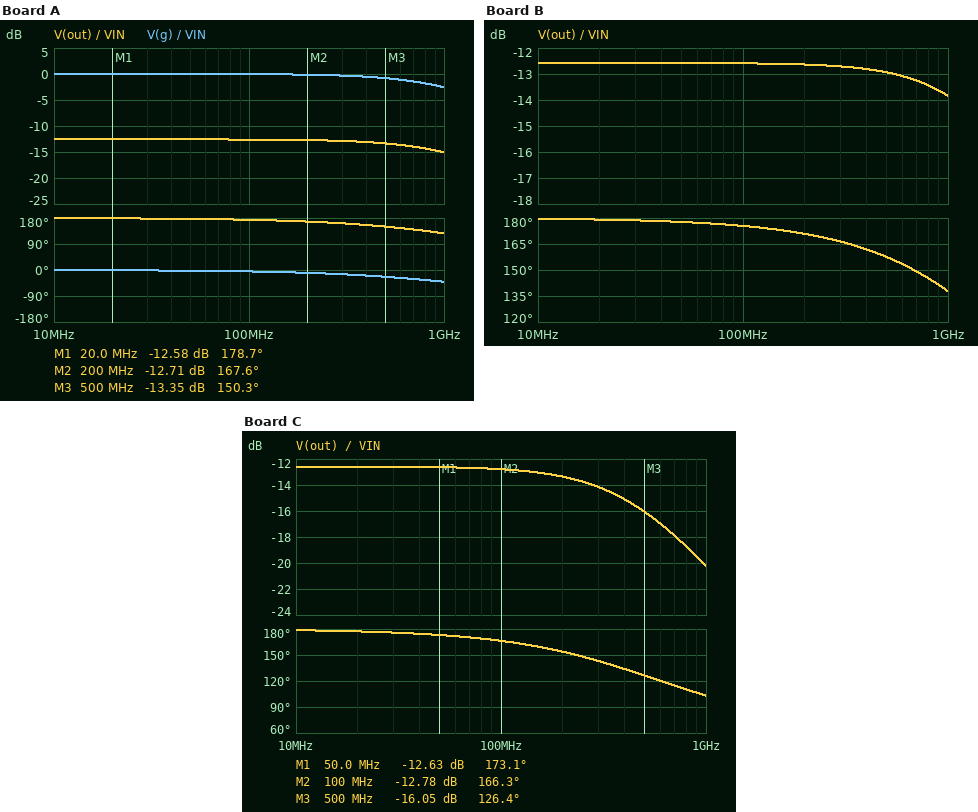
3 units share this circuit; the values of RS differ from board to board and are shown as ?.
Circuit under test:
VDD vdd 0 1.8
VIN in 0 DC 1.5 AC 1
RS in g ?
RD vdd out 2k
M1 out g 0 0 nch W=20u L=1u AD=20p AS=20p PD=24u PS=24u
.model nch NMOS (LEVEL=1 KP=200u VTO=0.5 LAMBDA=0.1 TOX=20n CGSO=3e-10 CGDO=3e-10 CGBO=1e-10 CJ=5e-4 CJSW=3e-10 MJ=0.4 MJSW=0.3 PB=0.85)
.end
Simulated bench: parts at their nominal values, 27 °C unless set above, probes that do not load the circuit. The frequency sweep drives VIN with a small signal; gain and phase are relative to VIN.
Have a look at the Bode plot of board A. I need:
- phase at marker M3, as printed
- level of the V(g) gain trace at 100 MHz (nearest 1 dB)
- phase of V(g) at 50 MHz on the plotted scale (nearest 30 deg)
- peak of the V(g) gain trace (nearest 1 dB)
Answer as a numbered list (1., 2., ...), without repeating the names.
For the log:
1. 150.3 deg
2. 0 dB
3. 0 deg
4. 0 dB
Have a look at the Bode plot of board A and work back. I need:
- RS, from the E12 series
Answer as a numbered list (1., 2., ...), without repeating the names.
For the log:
1. 2.7 kΩ
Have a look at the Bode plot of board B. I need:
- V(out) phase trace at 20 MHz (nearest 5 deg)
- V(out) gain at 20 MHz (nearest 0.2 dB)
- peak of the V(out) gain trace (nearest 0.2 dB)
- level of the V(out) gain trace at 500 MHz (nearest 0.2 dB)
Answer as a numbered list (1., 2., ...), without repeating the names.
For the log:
1. 180 deg
2. -12.6 dB
3. -12.6 dB
4. -13.0 dB
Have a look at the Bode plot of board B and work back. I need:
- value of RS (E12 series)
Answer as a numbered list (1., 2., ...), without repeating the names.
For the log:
1. 1.8 kΩ
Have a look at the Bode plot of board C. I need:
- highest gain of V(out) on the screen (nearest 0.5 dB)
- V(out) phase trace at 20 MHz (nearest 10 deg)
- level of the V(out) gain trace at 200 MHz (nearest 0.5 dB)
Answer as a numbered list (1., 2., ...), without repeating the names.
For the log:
1. -12.5 dB
2. 180 deg
3. -13.5 dB
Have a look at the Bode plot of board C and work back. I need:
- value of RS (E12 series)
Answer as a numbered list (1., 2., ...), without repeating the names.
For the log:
1. 6.8 kΩ
